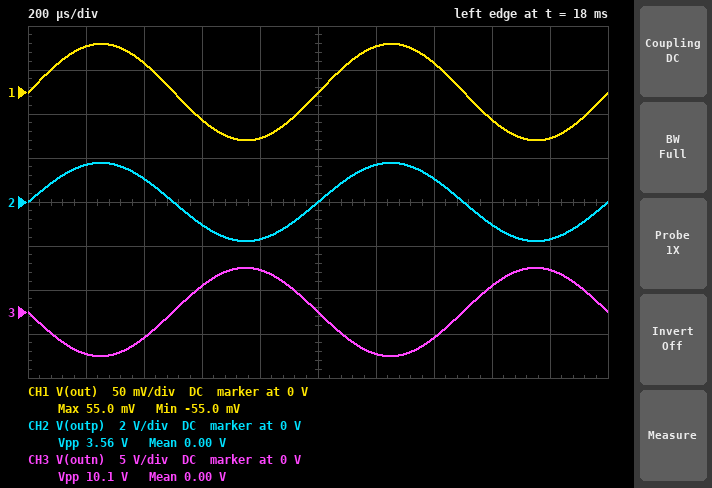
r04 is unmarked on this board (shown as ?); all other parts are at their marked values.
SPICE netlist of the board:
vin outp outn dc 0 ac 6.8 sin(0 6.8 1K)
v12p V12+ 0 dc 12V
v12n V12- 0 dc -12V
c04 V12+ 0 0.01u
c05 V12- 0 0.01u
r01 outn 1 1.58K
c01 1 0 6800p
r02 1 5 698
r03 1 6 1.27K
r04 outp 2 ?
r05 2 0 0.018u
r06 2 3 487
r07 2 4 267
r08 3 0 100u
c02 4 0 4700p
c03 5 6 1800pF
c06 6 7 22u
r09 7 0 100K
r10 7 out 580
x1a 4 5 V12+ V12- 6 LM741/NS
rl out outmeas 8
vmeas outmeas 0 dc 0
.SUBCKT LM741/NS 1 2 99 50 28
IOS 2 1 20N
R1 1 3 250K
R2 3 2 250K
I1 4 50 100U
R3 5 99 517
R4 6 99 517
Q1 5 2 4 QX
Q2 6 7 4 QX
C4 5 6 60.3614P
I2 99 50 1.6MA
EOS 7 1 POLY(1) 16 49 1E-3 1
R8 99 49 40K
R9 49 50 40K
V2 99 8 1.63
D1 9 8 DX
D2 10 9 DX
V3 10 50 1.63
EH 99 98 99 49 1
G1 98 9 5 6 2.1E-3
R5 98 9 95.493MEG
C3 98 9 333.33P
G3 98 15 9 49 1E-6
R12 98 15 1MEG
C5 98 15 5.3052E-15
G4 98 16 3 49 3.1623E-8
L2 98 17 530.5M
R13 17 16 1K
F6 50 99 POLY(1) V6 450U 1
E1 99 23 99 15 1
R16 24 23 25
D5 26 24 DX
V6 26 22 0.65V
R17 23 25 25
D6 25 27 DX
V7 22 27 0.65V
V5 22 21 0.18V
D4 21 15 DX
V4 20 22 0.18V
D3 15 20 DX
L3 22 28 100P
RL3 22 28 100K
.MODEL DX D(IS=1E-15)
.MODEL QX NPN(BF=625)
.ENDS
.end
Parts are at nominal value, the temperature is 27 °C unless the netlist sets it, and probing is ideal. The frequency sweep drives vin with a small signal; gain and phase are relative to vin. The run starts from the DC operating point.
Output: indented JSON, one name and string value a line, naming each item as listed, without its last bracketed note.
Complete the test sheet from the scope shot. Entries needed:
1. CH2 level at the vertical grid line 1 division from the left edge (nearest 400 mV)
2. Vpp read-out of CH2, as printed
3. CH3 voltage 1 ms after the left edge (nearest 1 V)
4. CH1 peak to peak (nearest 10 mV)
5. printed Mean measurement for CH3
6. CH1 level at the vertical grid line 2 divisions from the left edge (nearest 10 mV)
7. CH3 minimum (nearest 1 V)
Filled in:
{
  "CH2 level at the vertical grid line 1 division from the left edge": "1.6 V",
  "Vpp read-out of CH2, as printed": "3.56 V",
  "CH3 voltage 1 ms after the left edge": "0 V",
  "CH1 peak to peak": "110 mV",
  "printed Mean measurement for CH3": "0.00 V",
  "CH1 level at the vertical grid line 2 divisions from the left edge": "30 mV",
  "CH3 minimum": "-5 V"
}
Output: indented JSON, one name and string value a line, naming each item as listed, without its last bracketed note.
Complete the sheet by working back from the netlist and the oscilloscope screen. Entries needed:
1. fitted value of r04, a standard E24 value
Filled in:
{
  "fitted value of r04, a standard E24 value": "560 Ω"
}
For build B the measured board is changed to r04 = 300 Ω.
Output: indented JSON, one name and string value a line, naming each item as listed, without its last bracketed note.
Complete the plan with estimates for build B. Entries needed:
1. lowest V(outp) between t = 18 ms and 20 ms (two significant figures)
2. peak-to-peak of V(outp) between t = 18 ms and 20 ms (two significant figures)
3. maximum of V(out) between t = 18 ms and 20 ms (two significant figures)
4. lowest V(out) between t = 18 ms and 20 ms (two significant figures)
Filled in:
{
  "lowest V(outp) between t = 18 ms and 20 ms": "-1.1 V",
  "peak-to-peak of V(outp) between t = 18 ms and 20 ms": "2.2 V",
  "maximum of V(out) between t = 18 ms and 20 ms": "62 mV",
  "lowest V(out) between t = 18 ms and 20 ms": "-63 mV"
}
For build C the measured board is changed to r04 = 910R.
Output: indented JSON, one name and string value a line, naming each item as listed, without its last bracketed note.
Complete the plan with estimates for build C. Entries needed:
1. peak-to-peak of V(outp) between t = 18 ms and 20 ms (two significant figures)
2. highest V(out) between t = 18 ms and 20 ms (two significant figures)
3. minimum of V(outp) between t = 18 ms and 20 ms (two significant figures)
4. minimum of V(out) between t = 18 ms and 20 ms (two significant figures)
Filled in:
{
  "peak-to-peak of V(outp) between t = 18 ms and 20 ms": "5.0 V",
  "highest V(out) between t = 18 ms and 20 ms": "47 mV",
  "minimum of V(outp) between t = 18 ms and 20 ms": "-2.5 V",
  "minimum of V(out) between t = 18 ms and 20 ms": "-47 mV"
}
